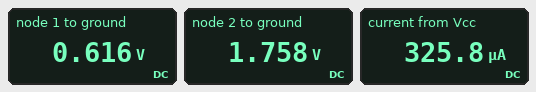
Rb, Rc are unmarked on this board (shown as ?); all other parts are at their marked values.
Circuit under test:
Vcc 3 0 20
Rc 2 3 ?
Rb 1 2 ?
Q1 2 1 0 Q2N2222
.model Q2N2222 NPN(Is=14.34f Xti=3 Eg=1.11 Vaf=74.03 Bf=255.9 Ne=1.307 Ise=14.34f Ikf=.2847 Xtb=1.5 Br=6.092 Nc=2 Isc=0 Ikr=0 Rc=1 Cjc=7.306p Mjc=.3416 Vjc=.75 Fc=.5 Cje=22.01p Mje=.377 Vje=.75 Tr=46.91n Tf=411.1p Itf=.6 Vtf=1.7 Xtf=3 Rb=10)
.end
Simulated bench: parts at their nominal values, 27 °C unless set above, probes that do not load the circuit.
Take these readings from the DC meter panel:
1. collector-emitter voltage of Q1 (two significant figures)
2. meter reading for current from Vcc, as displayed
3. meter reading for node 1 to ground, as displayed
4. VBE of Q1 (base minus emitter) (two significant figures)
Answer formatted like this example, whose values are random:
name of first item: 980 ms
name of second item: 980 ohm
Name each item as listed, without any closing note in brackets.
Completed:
collector-emitter voltage of Q1: 1.8 V
meter reading for current from Vcc, as displayed: 325.8 µA
meter reading for node 1 to ground, as displayed: 0.616 V
VBE of Q1 (base minus emitter): 620 mV
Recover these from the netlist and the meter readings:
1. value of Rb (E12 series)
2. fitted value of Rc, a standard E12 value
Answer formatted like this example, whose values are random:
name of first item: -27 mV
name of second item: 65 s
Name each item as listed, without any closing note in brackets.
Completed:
value of Rb: 470 kΩ
fitted value of Rc, a standard E12 value: 56 kΩ
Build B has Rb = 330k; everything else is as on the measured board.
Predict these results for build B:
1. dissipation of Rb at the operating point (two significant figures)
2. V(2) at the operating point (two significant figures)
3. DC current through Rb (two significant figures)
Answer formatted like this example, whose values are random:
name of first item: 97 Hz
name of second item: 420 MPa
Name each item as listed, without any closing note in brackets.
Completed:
dissipation of Rb at the operating point: 2.0 µW
V(2) at the operating point: 1.4 V
DC current through Rb: 2.5 µA
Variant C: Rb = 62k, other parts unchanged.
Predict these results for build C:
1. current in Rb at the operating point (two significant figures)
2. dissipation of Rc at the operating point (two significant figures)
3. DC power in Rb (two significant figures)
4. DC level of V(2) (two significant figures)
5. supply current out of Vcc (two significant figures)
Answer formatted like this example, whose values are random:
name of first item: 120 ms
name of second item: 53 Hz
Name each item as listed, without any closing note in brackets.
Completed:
current in Rb at the operating point: 2.6 µA
dissipation of Rc at the operating point: 6.6 mW
DC power in Rb: 410 nW
DC level of V(2): 780 mV
supply current out of Vcc: 340 µA
